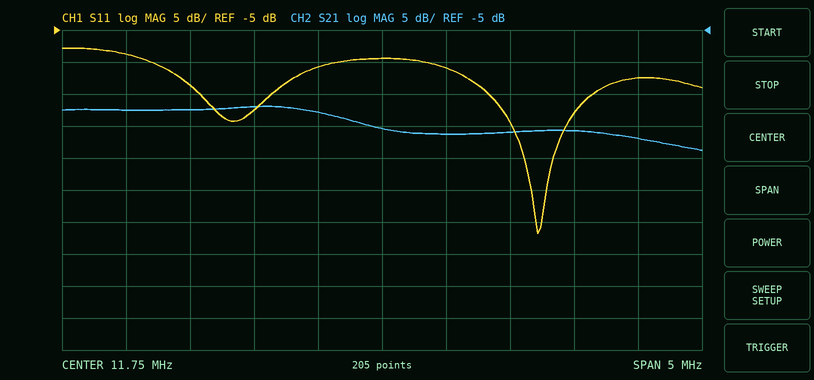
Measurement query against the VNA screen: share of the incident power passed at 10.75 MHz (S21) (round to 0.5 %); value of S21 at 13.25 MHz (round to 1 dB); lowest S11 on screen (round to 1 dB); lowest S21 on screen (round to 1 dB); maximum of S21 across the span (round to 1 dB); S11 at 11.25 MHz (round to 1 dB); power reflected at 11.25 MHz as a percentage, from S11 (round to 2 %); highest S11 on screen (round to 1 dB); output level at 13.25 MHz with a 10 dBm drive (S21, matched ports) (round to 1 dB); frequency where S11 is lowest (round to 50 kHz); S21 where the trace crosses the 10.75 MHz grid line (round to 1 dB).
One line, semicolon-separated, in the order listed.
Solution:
2.0 %; -21 dB; -37 dB; -24 dB; -17 dB; -11 dB; 8 %; -8 dB; -11 dBm; 12.95 MHz; -17 dB
